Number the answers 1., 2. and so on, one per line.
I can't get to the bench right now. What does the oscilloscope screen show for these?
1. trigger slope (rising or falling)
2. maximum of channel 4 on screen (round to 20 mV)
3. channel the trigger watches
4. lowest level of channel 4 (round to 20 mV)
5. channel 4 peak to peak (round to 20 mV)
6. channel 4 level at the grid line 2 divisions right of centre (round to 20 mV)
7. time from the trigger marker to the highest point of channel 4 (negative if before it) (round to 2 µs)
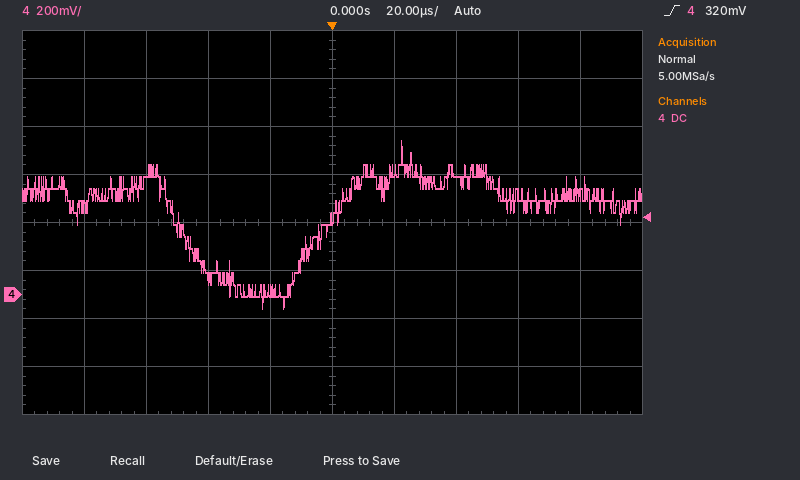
1. rising
2. 640 mV
3. channel 4
4. -60 mV
5. 700 mV
6. 500 mV
7. +22 µs
